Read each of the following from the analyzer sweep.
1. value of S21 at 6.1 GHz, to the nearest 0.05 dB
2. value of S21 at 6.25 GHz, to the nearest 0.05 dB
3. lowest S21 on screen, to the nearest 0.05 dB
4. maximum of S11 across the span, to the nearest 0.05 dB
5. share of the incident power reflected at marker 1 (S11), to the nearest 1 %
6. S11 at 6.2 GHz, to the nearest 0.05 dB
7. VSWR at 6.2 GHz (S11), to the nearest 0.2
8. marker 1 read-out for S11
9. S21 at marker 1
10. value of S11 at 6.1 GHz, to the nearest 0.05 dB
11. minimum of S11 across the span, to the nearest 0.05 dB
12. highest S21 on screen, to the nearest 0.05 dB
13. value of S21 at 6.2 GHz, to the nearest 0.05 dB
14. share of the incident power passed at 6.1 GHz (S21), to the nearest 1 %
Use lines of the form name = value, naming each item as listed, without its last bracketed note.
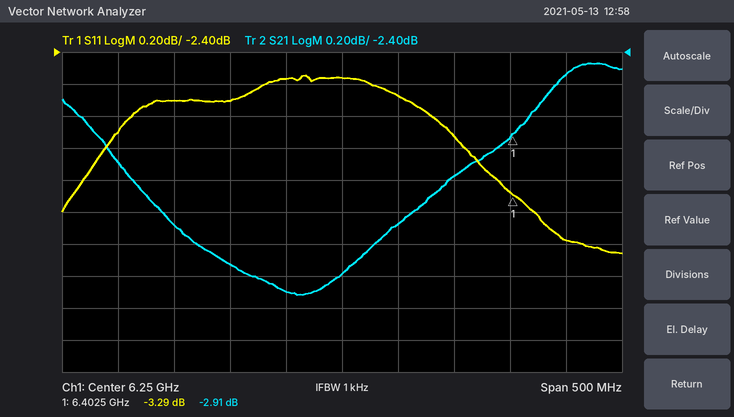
value of S21 at 6.1 GHz, to the nearest 0.05 dB = -3.50 dB
value of S21 at 6.25 GHz, to the nearest 0.05 dB = -3.80 dB
lowest S21 on screen, to the nearest 0.05 dB = -3.90 dB
maximum of S11 across the span, to the nearest 0.05 dB = -2.55 dB
share of the incident power reflected at marker 1 (S11), to the nearest 1 % = 47 %
S11 at 6.2 GHz, to the nearest 0.05 dB = -2.55 dB
VSWR at 6.2 GHz (S11), to the nearest 0.2 = 6.8
marker 1 read-out for S11 = -3.29 dB
S21 at marker 1 = -2.91 dB
value of S11 at 6.1 GHz, to the nearest 0.05 dB = -2.70 dB
minimum of S11 across the span, to the nearest 0.05 dB = -3.65 dB
highest S21 on screen, to the nearest 0.05 dB = -2.45 dB
value of S21 at 6.2 GHz, to the nearest 0.05 dB = -3.90 dB
share of the incident power passed at 6.1 GHz (S21), to the nearest 1 % = 45 %
